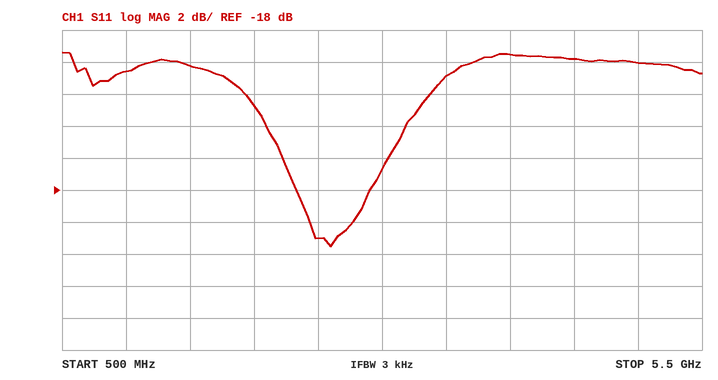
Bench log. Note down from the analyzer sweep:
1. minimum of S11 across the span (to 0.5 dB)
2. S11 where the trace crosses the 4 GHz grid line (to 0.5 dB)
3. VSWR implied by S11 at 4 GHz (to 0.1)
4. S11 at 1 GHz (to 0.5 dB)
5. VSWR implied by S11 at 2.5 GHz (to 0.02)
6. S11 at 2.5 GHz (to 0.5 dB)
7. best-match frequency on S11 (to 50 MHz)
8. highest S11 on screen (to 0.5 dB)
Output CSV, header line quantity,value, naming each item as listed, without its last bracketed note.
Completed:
quantity,value
minimum of S11 across the span,-21.5 dB
S11 where the trace crosses the 4 GHz grid line,-9.5 dB
VSWR implied by S11 at 4 GHz,2.0
S11 at 1 GHz,-10.5 dB
VSWR implied by S11 at 2.5 GHz,1.20
S11 at 2.5 GHz,-21.0 dB
best-match frequency on S11,2.60 GHz
highest S11 on screen,-9.5 dB
